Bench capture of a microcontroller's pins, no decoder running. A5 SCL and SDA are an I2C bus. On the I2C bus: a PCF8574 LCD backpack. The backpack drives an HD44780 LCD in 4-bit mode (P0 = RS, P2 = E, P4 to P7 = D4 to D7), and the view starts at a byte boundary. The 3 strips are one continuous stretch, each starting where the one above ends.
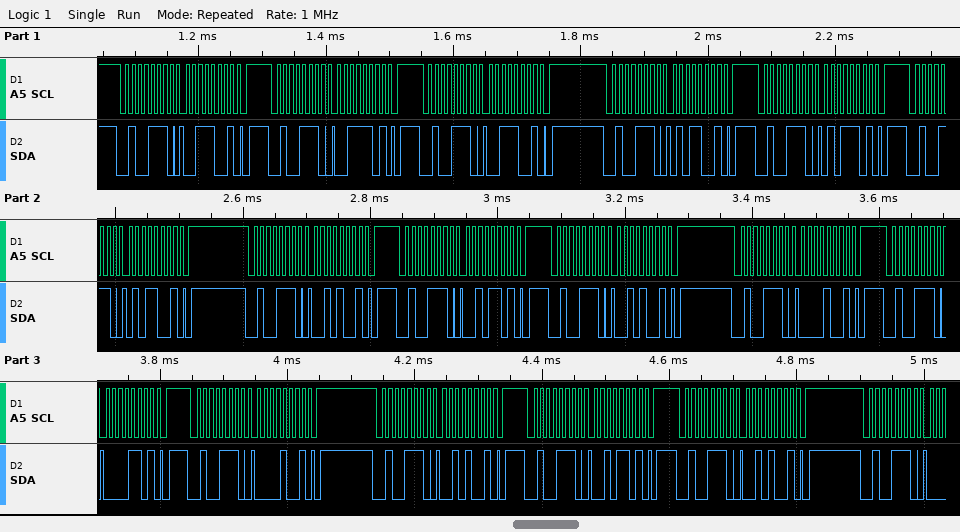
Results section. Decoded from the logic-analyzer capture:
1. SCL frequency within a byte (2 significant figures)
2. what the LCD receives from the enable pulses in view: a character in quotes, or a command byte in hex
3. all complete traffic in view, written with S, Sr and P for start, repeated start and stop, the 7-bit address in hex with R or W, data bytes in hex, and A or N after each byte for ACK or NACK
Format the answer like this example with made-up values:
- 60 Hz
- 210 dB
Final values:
- 100 kHz
- '5' ' '
- S 27W A 39 A P S 27W A 3D A P S 27W A 39 A P S 27W A 59 A P S 27W A 5D A P S 27W A 59 A P S 27W A 29 A P S 27W A 2D A P S 27W A 29 A P S 27W A 09 A P S 27W A 0D A P S 27W A 09 A P S 27W A 29 A P S 27W A 2D A P S 27W A 29 A P S 27W A
